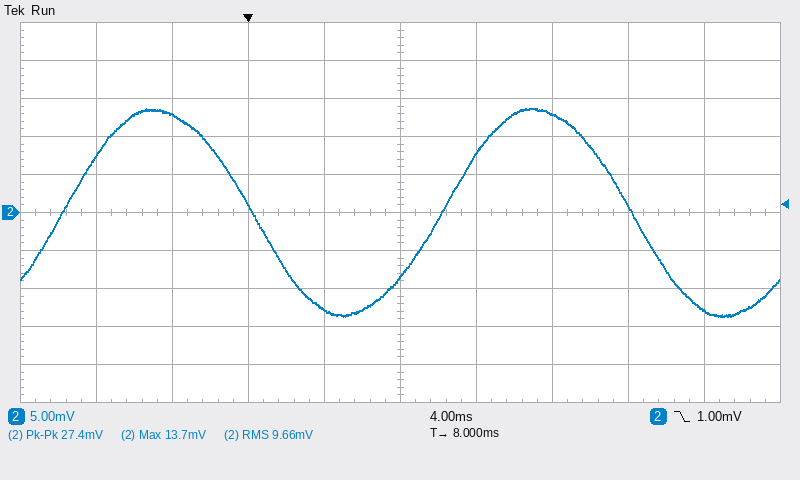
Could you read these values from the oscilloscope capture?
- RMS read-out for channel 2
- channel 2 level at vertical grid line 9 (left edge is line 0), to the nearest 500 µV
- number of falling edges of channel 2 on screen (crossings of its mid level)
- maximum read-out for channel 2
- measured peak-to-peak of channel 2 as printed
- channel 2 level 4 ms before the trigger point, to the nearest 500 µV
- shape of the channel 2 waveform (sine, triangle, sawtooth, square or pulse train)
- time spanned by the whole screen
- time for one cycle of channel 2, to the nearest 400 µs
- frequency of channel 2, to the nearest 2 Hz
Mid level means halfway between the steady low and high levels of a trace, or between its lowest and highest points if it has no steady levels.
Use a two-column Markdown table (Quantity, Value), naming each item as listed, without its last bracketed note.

| Quantity | Value |
|---|---|
| RMS read-out for channel 2 | 9.66 mV |
| channel 2 level at vertical grid line 9 (left edge is line 0), to the nearest 500 µV | -13.0 mV |
| number of falling edges of channel 2 on screen | 2 |
| maximum read-out for channel 2 | 13.7 mV |
| measured peak-to-peak of channel 2 as printed | 27.4 mV |
| channel 2 level 4 ms before the trigger point, to the nearest 500 µV | 13.0 mV |
| shape of the channel 2 waveform | sine |
| time spanned by the whole screen | 40 ms |
| time for one cycle of channel 2, to the nearest 400 µs | 20.0 ms |
| frequency of channel 2, to the nearest 2 Hz | 50 Hz |
